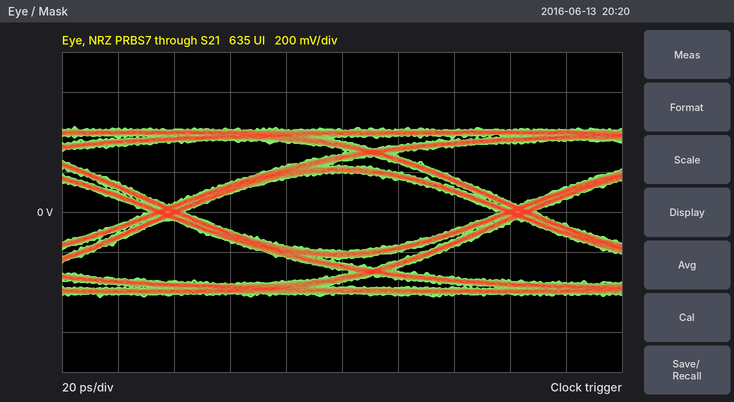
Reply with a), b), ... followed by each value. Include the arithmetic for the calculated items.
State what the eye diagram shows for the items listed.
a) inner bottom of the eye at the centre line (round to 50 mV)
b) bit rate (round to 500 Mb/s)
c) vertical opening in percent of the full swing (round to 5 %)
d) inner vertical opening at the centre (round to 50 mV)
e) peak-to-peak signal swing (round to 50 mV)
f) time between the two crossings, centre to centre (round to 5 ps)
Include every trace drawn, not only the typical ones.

a) -200 mV
b) 8.0 Gb/s
c) 400 mV / 850 mV ≈ 47.1 %, so 45 % to the nearest 5 %
d) 400 mV
e) 850 mV
f) 125 ps
